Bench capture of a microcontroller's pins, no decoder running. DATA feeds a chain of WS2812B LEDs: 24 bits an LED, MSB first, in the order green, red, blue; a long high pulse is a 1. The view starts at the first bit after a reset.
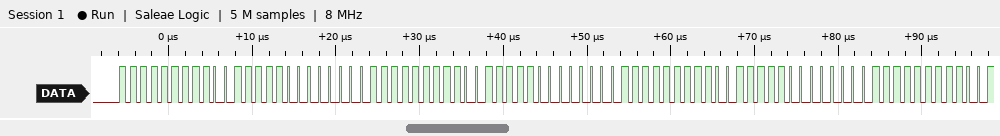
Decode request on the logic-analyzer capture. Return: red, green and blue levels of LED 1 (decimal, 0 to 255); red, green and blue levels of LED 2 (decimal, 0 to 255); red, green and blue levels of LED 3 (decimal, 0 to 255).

159, 255, 0
159, 255, 0
159, 255, 0
